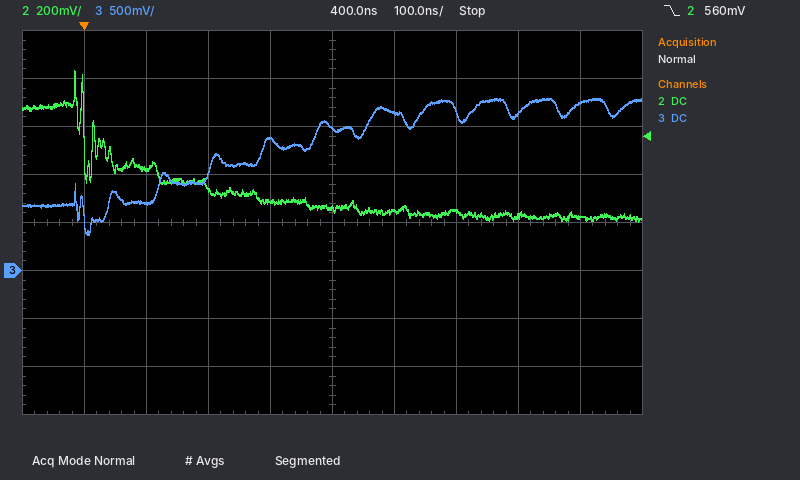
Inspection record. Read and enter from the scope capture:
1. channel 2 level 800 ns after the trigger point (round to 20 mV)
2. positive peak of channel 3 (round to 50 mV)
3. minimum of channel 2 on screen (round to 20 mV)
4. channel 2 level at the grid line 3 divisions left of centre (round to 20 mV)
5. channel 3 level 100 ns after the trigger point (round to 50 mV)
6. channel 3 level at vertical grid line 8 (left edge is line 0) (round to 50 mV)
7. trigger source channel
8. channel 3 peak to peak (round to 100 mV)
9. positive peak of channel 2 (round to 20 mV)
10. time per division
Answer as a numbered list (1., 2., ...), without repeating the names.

1. 220 mV
2. 1.80 V
3. 200 mV
4. 420 mV
5. 700 mV
6. 1.65 V
7. channel 2
8. 1.40 V
9. 840 mV
10. 100 ns
